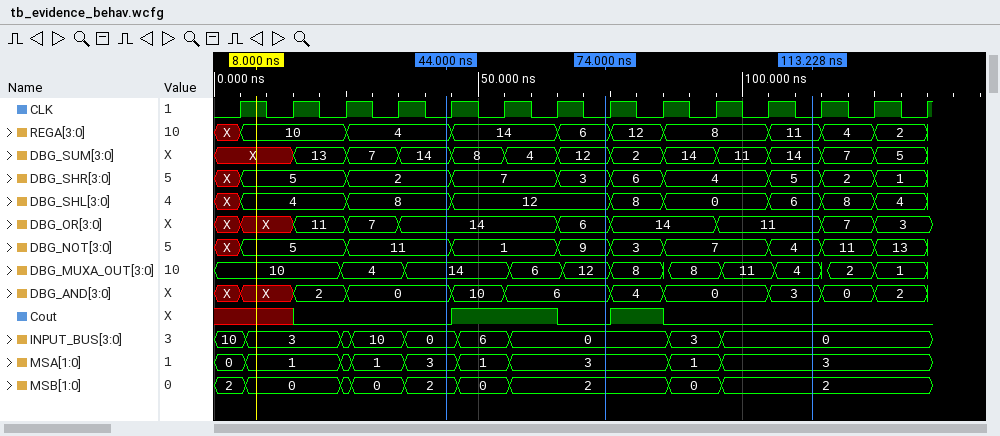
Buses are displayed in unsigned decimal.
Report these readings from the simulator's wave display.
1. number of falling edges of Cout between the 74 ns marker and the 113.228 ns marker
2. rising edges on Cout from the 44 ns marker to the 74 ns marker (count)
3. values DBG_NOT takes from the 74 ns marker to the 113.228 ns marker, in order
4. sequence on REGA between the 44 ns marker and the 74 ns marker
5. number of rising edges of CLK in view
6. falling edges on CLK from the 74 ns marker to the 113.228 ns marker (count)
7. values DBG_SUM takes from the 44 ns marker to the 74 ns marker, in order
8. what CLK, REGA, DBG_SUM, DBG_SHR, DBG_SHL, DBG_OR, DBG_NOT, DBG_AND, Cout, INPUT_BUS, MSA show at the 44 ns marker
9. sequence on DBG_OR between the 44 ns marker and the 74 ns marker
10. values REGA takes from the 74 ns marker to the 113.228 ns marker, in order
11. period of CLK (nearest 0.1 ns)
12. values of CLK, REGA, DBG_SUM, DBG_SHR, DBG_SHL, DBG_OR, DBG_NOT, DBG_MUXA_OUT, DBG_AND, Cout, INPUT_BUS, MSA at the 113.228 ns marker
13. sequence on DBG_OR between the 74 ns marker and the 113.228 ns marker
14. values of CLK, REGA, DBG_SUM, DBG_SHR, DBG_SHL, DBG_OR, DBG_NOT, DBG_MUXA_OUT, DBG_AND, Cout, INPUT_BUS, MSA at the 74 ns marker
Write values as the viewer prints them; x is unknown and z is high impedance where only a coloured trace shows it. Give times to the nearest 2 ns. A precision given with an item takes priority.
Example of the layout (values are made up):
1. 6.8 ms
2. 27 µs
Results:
1. 1
2. 1
3. 9, 3, 7, 4
4. 4, 14, 6
5. 14
6. 4
7. 14, 8, 4, 12
8. CLK=0, REGA=4, DBG_SUM=14, DBG_SHR=2, DBG_SHL=8, DBG_OR=14, DBG_NOT=11, DBG_AND=0, Cout=0, INPUT_BUS=0, MSA=3
9. 14, 6
10. 6, 12, 8, 11
11. 10 ns
12. CLK=0, REGA=11, DBG_SUM=14, DBG_SHR=5, DBG_SHL=6, DBG_OR=11, DBG_NOT=4, DBG_MUXA_OUT=4, DBG_AND=3, Cout=0, INPUT_BUS=0, MSA=3
13. 6, 14, 11
14. CLK=0, REGA=6, DBG_SUM=12, DBG_SHR=3, DBG_SHL=12, DBG_OR=6, DBG_NOT=9, DBG_MUXA_OUT=12, DBG_AND=6, Cout=0, INPUT_BUS=0, MSA=3
